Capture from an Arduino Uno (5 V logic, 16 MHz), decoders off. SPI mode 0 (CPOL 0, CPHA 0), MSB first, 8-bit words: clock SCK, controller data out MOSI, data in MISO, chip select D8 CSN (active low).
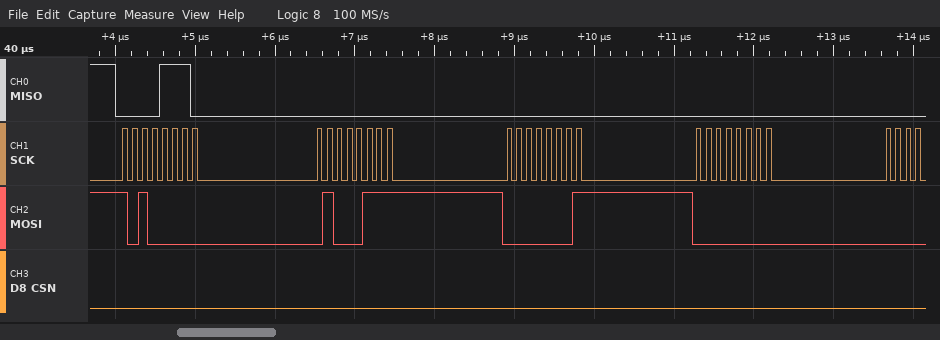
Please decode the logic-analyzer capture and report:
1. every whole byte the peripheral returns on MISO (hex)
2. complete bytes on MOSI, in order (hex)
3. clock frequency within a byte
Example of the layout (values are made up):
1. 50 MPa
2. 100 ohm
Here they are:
1. 0E 00 00 00
2. A0 47 01 00
3. 8 MHz
